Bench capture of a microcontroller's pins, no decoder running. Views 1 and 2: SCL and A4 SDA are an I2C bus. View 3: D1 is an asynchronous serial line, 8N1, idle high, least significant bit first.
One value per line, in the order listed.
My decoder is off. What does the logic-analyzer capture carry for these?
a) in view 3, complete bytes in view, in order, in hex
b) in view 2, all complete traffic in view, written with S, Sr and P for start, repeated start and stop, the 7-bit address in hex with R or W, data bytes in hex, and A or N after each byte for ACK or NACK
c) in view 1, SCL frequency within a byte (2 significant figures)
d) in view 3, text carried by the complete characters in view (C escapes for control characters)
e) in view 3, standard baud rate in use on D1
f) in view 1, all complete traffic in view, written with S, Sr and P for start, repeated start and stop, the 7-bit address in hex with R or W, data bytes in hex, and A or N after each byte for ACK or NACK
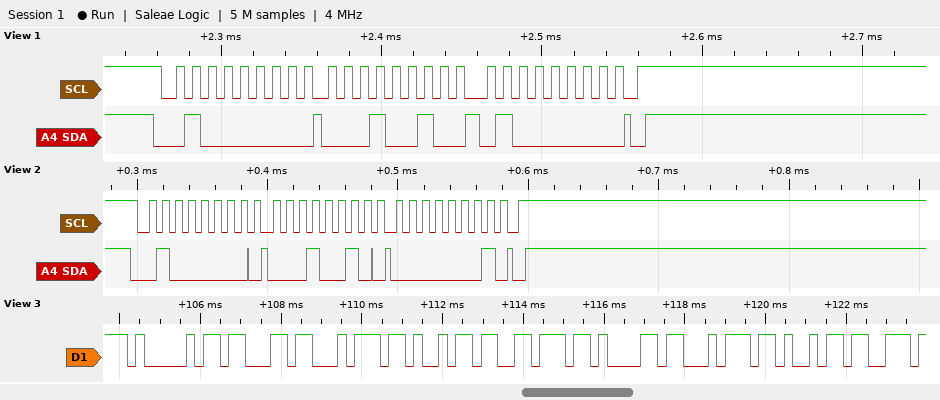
41 63 74 69 76 61 74 69
S 20W A 12 A 01 A P
100 kHz
"Activati"
4800 baud
S 20W A 12 A 40 A P
